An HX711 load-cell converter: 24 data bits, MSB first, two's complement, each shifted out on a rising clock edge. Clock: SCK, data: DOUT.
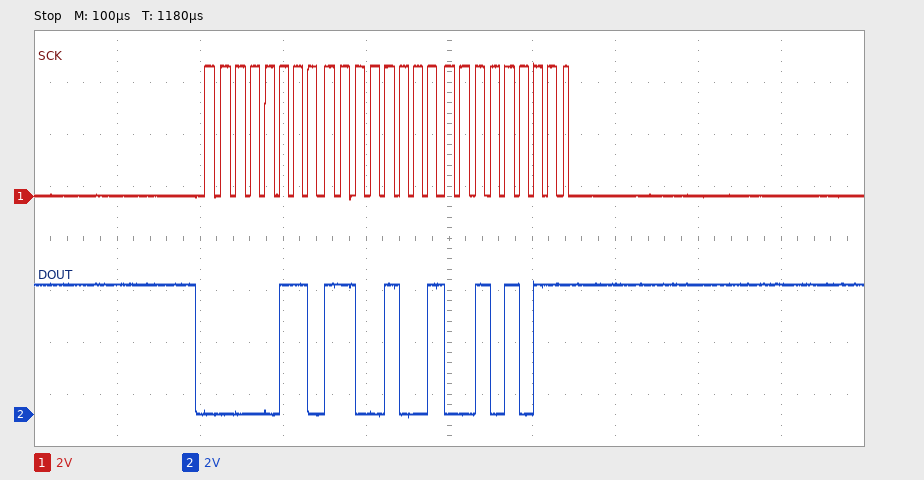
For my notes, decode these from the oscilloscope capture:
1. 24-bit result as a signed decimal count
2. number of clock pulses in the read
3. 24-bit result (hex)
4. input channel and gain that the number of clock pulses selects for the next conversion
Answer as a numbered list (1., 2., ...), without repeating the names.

1. 444715
2. 25
3. 0x06C92B
4. channel A, gain 128
